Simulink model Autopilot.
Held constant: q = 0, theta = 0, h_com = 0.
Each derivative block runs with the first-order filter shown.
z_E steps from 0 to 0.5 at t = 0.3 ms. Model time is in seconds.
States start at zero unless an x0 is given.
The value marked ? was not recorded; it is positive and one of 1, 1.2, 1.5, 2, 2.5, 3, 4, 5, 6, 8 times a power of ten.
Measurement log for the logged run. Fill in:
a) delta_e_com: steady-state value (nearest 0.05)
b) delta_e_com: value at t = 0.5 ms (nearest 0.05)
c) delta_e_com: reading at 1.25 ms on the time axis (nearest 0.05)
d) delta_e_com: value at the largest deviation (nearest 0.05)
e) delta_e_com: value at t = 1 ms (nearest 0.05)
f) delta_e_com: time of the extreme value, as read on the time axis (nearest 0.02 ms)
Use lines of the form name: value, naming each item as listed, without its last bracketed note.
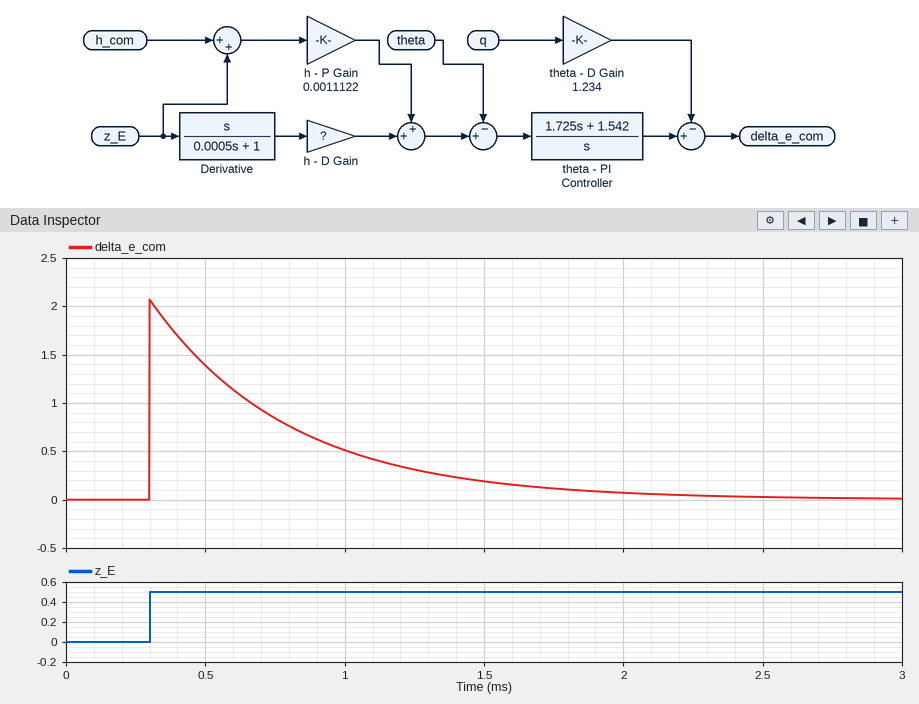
delta_e_com: steady-state value: 0.00
delta_e_com: value at t = 0.5 ms: 1.40
delta_e_com: reading at 1.25 ms on the time axis: 0.30
delta_e_com: value at the largest deviation: 2.05
delta_e_com: value at t = 1 ms: 0.50
delta_e_com: time of the extreme value, as read on the time axis: 0.30 ms
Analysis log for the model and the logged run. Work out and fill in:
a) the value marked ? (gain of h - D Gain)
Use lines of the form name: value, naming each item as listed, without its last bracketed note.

the value marked ?: 0.0012
